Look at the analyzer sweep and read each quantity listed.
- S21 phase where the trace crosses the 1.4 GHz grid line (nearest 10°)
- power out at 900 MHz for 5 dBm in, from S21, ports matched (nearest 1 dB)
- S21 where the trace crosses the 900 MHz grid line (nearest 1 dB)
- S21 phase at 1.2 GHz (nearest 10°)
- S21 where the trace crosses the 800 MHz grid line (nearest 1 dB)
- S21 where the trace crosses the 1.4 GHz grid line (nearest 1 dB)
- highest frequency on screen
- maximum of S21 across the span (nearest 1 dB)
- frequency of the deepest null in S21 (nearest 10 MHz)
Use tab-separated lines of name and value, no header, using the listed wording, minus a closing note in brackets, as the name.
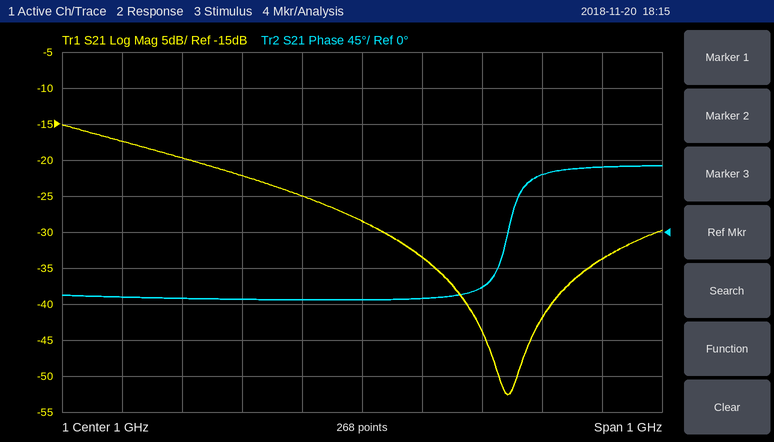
S21 phase where the trace crosses the 1.4 GHz grid line	80°
power out at 900 MHz for 5 dBm in, from S21, ports matched	-20 dBm
S21 where the trace crosses the 900 MHz grid line	-25 dB
S21 phase at 1.2 GHz	-70°
S21 where the trace crosses the 800 MHz grid line	-22 dB
S21 where the trace crosses the 1.4 GHz grid line	-34 dB
highest frequency on screen	1.5 GHz
maximum of S21 across the span	-15 dB
frequency of the deepest null in S21	1.24 GHz
